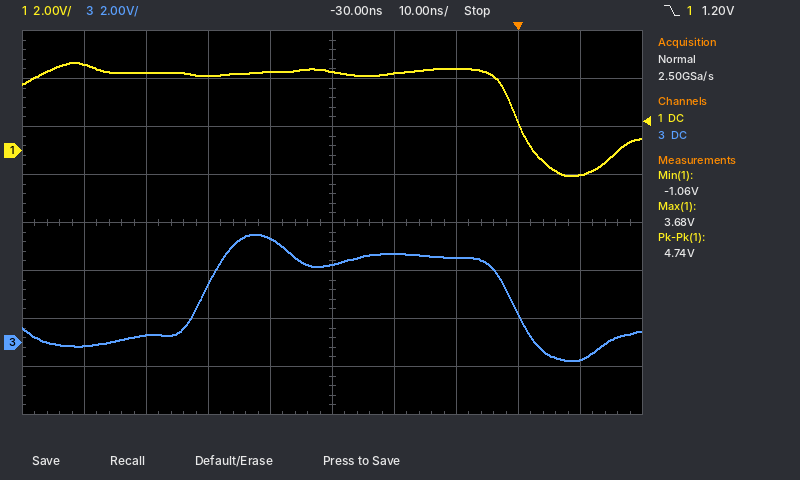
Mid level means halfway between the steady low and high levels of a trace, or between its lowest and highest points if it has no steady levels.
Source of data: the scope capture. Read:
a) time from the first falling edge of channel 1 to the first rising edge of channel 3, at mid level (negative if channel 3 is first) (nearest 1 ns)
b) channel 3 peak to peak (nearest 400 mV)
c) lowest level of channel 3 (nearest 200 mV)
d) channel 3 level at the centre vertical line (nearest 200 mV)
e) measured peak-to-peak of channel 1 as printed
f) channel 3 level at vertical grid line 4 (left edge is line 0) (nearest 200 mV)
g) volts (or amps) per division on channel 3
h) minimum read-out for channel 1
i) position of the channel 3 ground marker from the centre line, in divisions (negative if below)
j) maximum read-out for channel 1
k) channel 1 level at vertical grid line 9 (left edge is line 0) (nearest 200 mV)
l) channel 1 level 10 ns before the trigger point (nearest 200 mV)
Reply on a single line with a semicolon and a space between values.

-51 ns; 5.2 V; -800 mV; 3.2 V; 4.74 V; 4.4 V; 2 V; -1.06 V; -2.5 div; 3.68 V; -1.0 V; 3.4 V
